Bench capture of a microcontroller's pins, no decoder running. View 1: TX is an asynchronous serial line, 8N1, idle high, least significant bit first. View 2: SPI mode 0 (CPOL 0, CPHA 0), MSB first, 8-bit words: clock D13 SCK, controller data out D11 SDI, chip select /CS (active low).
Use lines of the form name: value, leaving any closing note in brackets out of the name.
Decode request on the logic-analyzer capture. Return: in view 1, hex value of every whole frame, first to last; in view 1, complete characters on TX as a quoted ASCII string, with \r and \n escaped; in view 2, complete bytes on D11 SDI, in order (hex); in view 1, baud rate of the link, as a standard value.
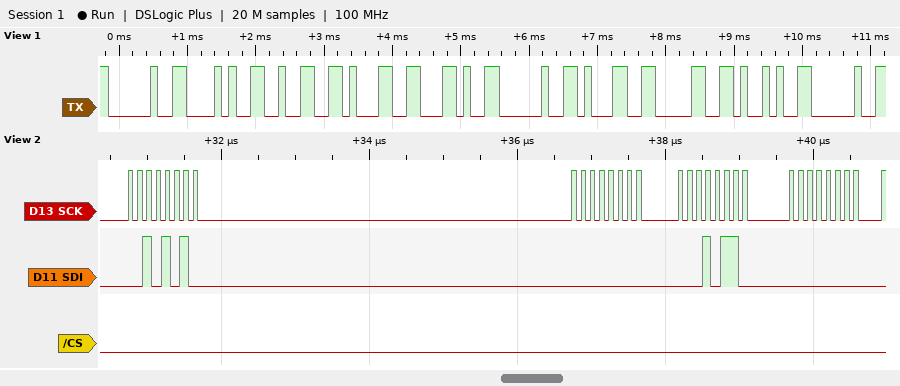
in view 1, hex value of every whole frame, first to last: 20 28 32 31 2C 20 31 30 29 20
in view 1, complete characters on TX as a quoted ASCII string, with \r and \n escaped: " (21, 10) "
in view 2, complete bytes on D11 SDI, in order: 2A 00 16 00
in view 1, baud rate of the link, as a standard value: 9600 baud
